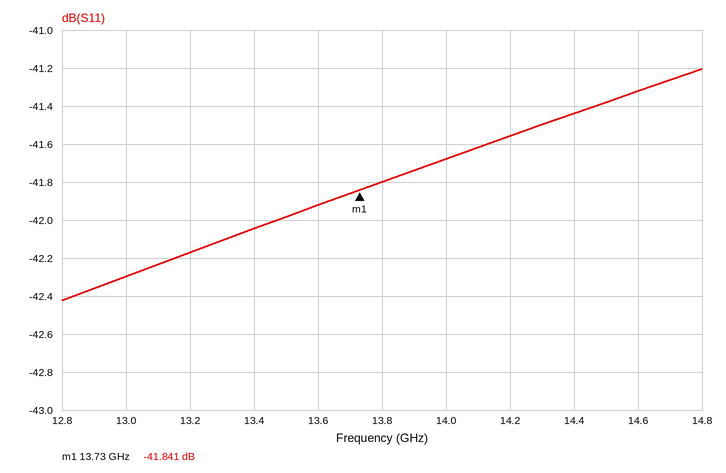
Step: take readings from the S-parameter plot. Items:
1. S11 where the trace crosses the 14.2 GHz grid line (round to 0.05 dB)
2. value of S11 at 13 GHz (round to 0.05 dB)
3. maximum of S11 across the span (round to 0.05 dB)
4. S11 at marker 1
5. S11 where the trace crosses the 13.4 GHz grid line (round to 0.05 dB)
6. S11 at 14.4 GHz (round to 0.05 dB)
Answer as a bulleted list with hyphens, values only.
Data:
- -41.55 dB
- -42.30 dB
- -41.20 dB
- -41.841 dB
- -42.05 dB
- -41.45 dB
